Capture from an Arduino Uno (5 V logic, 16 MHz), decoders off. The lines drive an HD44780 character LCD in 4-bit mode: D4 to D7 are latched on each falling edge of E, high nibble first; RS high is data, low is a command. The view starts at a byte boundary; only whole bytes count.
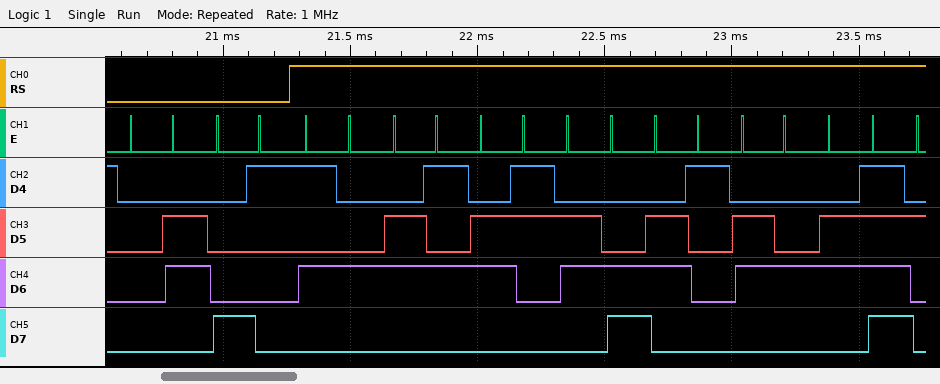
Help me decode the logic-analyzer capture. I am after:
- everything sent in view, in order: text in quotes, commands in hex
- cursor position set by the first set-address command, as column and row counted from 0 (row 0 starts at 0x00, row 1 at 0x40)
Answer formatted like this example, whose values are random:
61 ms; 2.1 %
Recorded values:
0x06 0x81 "Teclado"; column 1, row 0
